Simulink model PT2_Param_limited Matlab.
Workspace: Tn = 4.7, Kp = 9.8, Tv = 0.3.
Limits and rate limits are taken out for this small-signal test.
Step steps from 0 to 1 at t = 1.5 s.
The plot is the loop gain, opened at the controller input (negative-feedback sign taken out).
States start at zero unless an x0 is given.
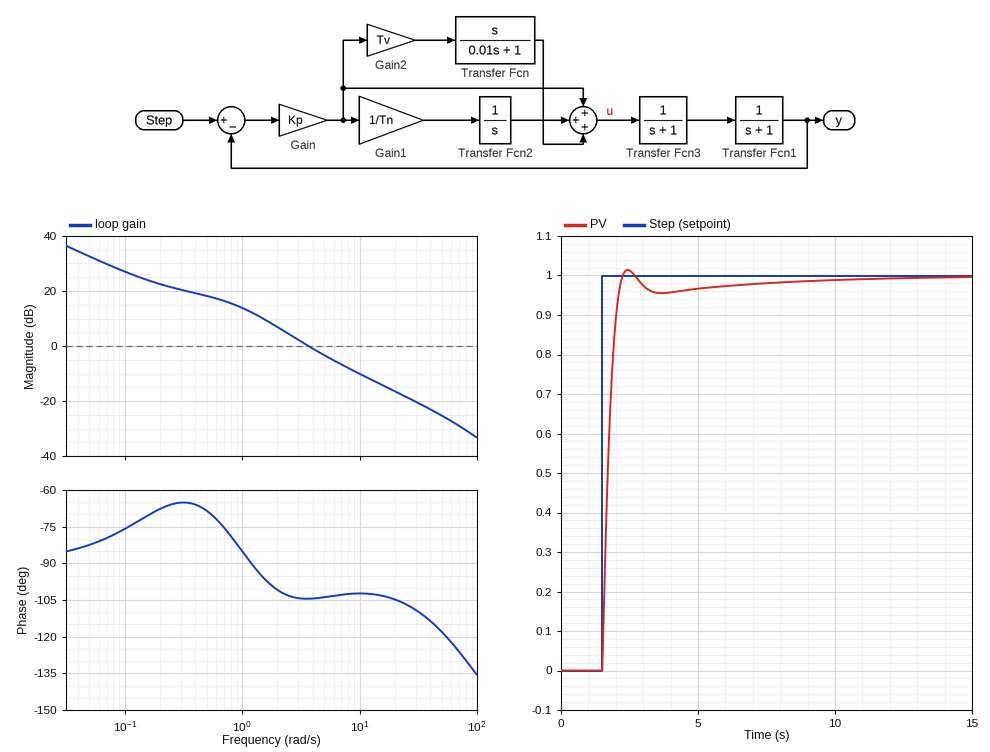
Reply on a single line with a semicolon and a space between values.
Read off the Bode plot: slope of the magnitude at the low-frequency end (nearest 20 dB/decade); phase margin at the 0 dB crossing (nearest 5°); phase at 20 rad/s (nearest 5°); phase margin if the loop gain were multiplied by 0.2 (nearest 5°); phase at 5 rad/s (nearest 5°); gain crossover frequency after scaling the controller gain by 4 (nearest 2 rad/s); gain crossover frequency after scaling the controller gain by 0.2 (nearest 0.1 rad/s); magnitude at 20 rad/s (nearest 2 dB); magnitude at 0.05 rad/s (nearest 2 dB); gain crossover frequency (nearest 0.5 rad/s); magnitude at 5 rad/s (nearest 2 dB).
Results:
-20 dB/decade; 75°; -105°; 95°; -105°; 12 rad/s; 1.0 rad/s; -16 dB; 32 dB; 3.5 rad/s; -4 dB
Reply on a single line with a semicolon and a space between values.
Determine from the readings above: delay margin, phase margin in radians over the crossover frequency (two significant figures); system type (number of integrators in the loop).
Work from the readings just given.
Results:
0.37 s; 1
